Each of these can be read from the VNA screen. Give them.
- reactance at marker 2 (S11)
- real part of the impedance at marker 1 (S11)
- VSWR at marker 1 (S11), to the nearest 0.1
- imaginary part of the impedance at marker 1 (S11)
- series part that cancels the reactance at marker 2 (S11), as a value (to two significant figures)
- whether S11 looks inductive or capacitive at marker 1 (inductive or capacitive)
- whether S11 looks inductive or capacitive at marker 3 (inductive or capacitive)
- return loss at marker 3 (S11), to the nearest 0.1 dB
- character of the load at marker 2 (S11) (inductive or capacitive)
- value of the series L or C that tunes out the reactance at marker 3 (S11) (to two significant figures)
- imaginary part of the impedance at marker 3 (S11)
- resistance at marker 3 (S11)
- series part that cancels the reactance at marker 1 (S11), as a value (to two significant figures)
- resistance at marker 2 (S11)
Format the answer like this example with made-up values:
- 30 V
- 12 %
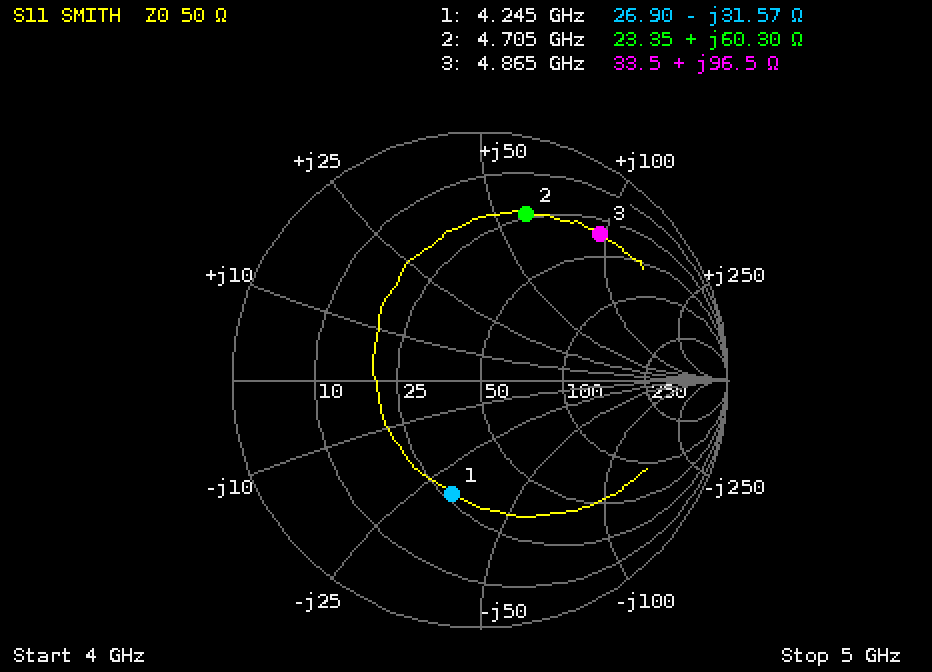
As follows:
- +60.30 Ω
- 26.90 Ω
- 2.8
- -31.57 Ω
- 560 fF
- capacitive
- inductive
- 2.3 dB
- inductive
- 340 fF
- +96.5 Ω
- 33.5 Ω
- 1.2 nH
- 23.35 Ω
